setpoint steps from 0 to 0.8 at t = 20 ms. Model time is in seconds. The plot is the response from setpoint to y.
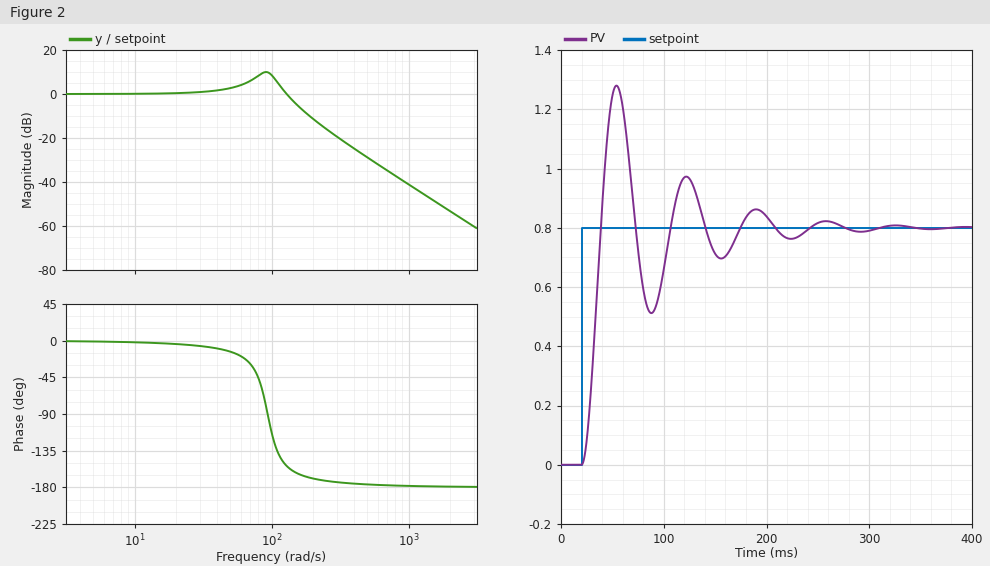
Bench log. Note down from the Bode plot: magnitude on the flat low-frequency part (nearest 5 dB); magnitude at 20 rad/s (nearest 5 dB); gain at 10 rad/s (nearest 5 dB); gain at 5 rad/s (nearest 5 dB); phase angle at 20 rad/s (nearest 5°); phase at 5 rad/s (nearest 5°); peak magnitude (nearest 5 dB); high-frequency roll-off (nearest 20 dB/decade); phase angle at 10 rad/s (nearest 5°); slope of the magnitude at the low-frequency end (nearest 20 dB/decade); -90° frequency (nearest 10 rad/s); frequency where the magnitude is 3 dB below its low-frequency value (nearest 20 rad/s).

0 dB
0 dB
0 dB
0 dB
-5°
0°
10 dB
-40 dB/decade
0°
0 dB/decade
90 rad/s
140 rad/s
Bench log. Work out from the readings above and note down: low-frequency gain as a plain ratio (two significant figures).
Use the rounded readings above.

1.0
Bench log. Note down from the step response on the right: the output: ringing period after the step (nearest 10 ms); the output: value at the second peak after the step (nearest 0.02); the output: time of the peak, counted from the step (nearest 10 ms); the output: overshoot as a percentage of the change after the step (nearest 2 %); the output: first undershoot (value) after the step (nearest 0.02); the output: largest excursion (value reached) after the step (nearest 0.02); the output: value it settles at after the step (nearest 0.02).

70 ms
0.98
30 ms
60 %
0.52
1.28
0.80
